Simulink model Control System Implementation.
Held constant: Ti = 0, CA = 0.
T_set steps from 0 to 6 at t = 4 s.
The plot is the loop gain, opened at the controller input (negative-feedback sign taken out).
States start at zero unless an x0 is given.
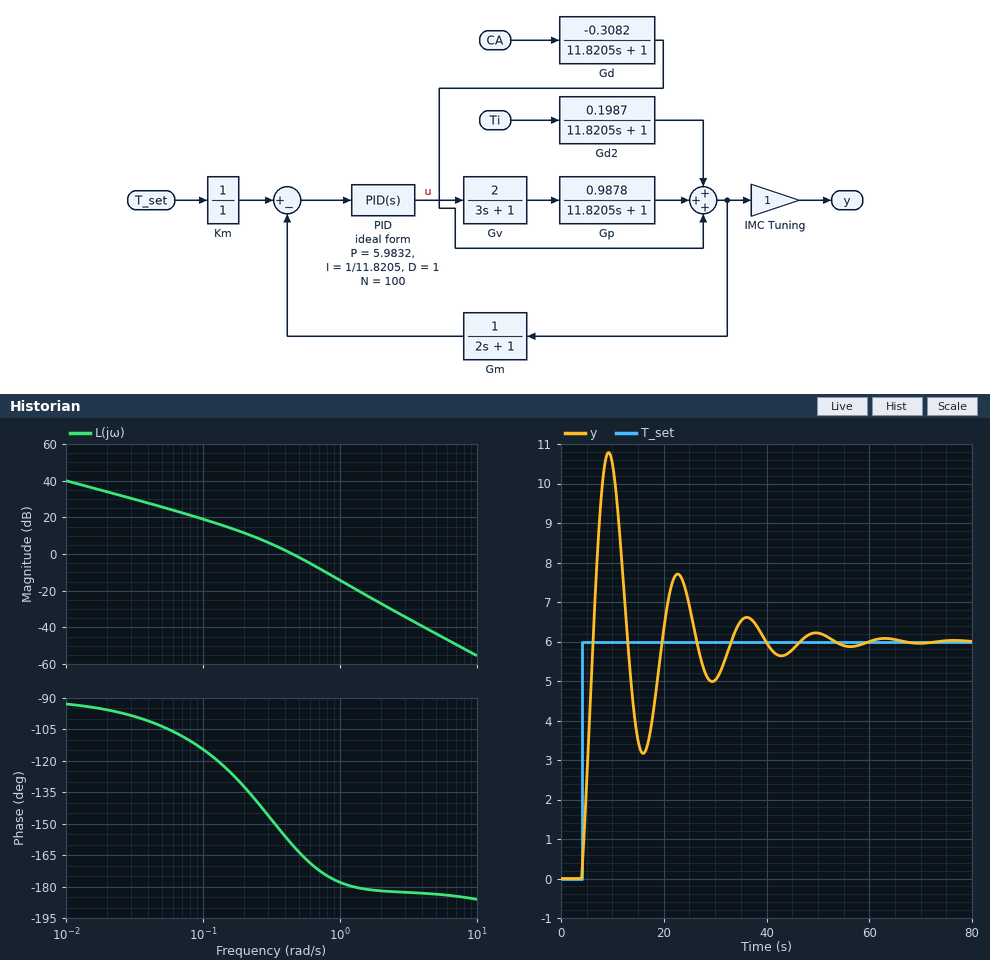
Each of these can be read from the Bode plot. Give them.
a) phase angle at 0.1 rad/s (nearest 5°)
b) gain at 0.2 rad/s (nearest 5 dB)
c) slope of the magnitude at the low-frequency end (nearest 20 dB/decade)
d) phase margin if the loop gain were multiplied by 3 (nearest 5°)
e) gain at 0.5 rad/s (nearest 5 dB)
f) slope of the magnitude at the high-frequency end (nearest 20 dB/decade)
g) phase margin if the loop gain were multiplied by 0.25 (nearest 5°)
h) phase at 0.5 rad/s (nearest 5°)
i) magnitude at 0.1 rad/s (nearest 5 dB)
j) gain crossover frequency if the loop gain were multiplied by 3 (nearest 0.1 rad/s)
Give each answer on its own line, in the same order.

-115°
10 dB
-20 dB/decade
5°
0 dB
-40 dB/decade
50°
-165°
20 dB
0.8 rad/s
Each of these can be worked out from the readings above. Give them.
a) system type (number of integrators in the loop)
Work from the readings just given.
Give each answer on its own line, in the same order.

1
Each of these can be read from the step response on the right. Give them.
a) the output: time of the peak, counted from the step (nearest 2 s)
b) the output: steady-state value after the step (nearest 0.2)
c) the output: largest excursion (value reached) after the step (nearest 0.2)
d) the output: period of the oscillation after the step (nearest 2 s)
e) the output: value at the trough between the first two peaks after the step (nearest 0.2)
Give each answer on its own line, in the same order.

6 s
6.0
10.8
14 s
3.2
